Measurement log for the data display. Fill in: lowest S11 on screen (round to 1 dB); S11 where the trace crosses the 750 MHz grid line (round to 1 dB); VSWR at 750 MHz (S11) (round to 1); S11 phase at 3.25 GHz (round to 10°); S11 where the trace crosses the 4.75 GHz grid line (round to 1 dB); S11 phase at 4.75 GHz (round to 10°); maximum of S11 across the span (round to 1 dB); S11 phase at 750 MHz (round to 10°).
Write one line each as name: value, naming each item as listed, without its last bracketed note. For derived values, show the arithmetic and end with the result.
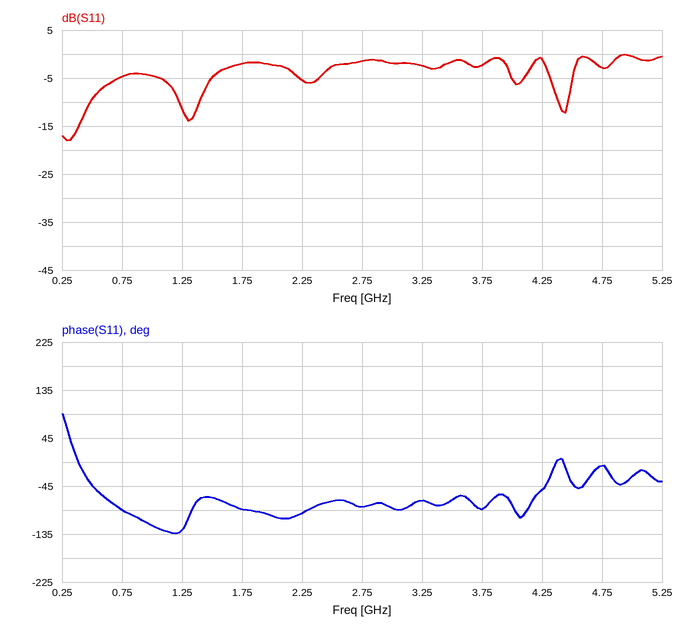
lowest S11 on screen: -18 dB
S11 where the trace crosses the 750 MHz grid line: -5 dB
VSWR at 750 MHz (S11): |Γ| = 10^(-5/20) = 0.5623; VSWR = (1 + 0.5623)/(1 − 0.5623) ≈ 4
S11 phase at 3.25 GHz: -70°
S11 where the trace crosses the 4.75 GHz grid line: -3 dB
S11 phase at 4.75 GHz: -10°
maximum of S11 across the span: 0 dB
S11 phase at 750 MHz: -90°
